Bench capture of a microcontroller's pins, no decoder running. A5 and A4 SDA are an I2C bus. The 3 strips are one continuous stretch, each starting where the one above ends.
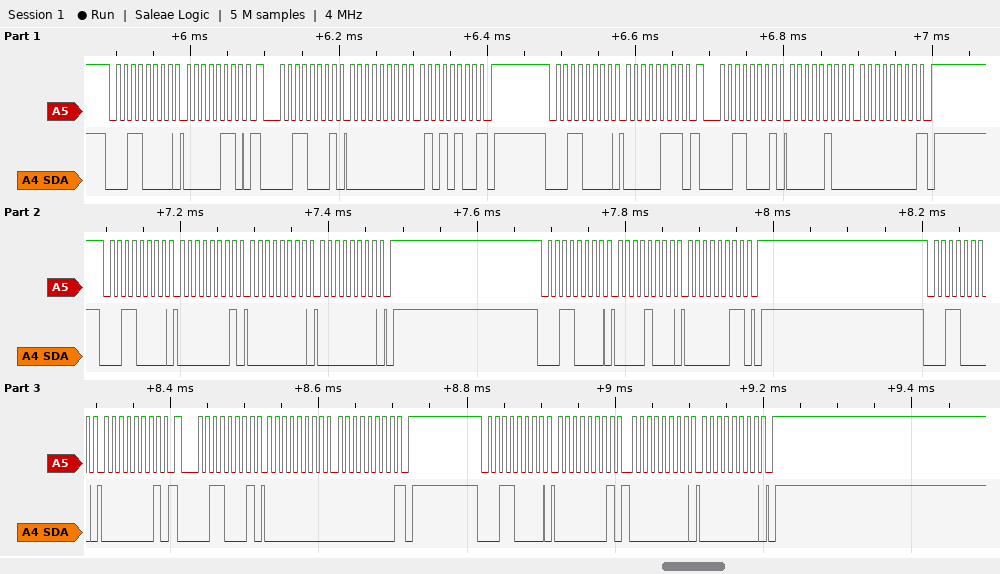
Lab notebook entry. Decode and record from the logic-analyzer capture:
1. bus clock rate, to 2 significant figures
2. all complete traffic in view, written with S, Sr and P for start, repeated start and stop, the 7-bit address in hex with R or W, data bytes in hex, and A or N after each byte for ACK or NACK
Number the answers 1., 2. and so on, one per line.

1. 100 kHz
2. S 18W A 06 A Sr 18R A 00 A 54 N P S 18W A 07 A Sr 18R A 04 A 00 N P S 18W A 01 A 00 A 00 A P S 18W A 08 A 03 A P S 18W A 01 A Sr 18R A 00 A 00 N P S 18W A 01 A 00 A 00 A P
